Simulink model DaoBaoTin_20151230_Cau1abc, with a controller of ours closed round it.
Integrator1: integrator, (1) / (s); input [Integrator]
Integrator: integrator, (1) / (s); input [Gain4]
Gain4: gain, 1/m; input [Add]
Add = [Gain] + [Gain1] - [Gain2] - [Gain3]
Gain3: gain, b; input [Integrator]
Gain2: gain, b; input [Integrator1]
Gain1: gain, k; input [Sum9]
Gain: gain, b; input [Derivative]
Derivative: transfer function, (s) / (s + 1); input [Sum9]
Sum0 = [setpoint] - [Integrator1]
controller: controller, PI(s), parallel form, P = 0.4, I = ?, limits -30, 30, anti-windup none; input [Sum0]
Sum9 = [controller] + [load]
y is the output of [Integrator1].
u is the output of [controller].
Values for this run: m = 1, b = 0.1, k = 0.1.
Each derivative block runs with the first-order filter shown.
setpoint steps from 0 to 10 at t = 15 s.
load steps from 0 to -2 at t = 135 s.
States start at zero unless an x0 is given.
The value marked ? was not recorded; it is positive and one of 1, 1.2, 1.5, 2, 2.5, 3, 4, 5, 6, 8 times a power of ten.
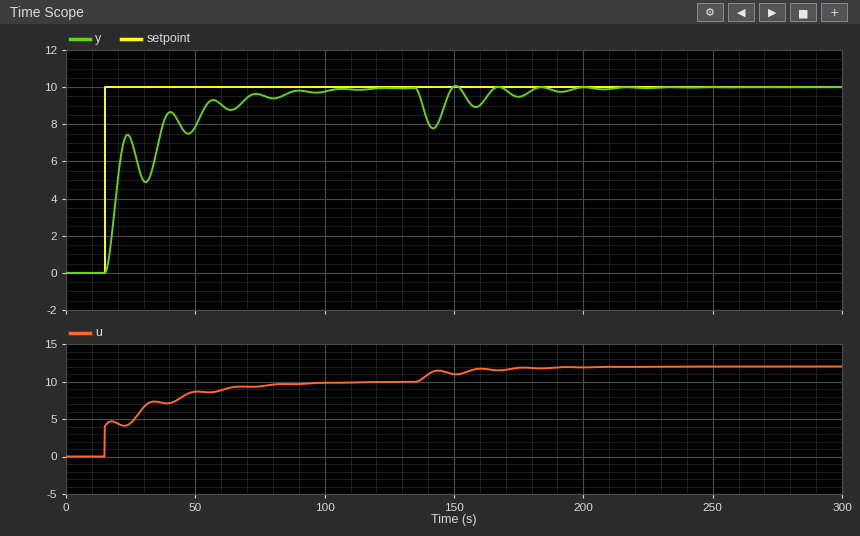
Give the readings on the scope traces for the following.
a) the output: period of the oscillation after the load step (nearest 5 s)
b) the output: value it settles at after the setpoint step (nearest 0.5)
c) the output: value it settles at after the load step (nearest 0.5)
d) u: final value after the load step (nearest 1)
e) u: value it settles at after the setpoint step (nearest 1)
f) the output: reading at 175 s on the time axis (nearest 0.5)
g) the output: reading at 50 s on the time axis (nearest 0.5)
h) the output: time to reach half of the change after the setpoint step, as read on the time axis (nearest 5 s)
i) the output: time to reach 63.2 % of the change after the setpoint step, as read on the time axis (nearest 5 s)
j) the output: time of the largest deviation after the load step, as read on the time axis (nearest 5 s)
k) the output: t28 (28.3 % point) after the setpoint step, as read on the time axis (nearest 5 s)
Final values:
15 s
10.0
10.0
12
10
9.5
8.0
20 s
20 s
140 s
20 s
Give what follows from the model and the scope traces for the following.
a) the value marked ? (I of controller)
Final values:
0.06
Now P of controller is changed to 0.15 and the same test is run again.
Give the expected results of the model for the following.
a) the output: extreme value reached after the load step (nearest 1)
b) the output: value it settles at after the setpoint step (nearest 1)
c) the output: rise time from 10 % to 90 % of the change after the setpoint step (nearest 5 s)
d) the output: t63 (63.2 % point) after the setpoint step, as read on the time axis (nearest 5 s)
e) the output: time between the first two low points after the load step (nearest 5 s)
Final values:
7
10
25 s
25 s
20 s
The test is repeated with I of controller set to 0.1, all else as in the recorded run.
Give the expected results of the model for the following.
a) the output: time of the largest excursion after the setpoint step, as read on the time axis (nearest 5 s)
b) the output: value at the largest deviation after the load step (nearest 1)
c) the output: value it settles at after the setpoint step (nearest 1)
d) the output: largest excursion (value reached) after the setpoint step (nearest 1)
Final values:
55 s
8
10
11
